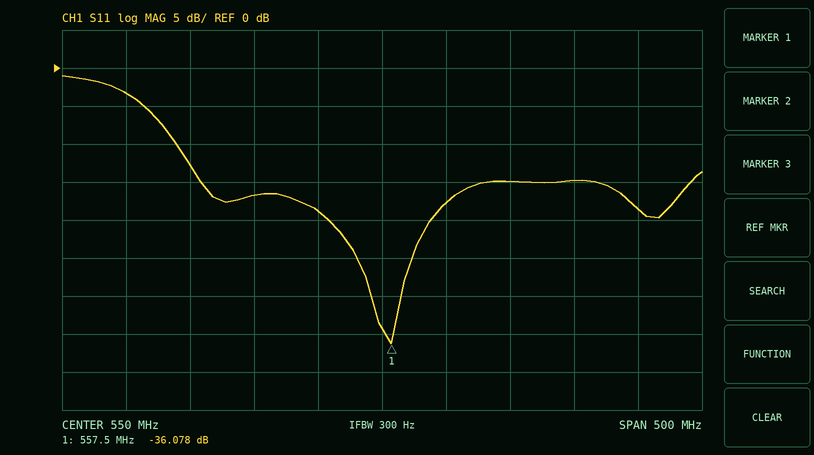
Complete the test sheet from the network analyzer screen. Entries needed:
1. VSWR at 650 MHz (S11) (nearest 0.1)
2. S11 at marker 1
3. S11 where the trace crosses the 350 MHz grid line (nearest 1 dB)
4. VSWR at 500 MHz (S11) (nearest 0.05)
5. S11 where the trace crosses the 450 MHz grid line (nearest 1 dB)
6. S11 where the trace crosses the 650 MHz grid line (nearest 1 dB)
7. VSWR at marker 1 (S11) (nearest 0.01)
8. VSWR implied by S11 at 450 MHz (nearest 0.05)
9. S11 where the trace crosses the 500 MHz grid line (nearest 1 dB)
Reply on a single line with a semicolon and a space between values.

1.4; -36.078 dB; -3 dB; 1.25; -17 dB; -15 dB; 1.03; 1.35; -19 dB
